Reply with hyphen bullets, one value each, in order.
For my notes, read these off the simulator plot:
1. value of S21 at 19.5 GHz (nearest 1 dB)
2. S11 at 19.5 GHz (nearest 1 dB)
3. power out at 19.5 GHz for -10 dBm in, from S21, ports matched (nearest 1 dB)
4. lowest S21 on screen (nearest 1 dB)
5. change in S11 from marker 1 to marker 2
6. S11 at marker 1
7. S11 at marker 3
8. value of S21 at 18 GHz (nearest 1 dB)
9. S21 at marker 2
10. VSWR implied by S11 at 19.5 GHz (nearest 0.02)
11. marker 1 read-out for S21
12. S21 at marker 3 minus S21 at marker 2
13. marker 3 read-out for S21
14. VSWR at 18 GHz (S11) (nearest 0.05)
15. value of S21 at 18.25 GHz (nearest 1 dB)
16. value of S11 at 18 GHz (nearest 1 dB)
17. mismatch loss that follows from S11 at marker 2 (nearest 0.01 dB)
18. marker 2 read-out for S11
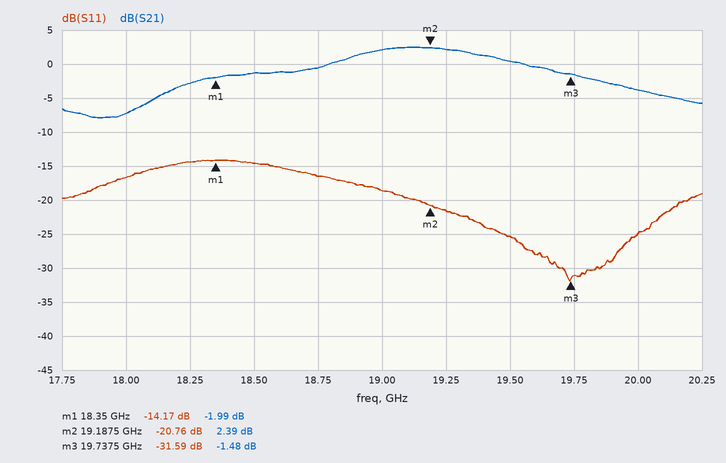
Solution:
- 0 dB
- -25 dB
- -10 dBm
- -8 dB
- -6.59 dB
- -14.17 dB
- -31.59 dB
- -7 dB
- 2.39 dB
- 1.12
- -1.99 dB
- -3.87 dB
- -1.48 dB
- 1.35
- -3 dB
- -17 dB
- 0.04 dB
- -20.76 dB
